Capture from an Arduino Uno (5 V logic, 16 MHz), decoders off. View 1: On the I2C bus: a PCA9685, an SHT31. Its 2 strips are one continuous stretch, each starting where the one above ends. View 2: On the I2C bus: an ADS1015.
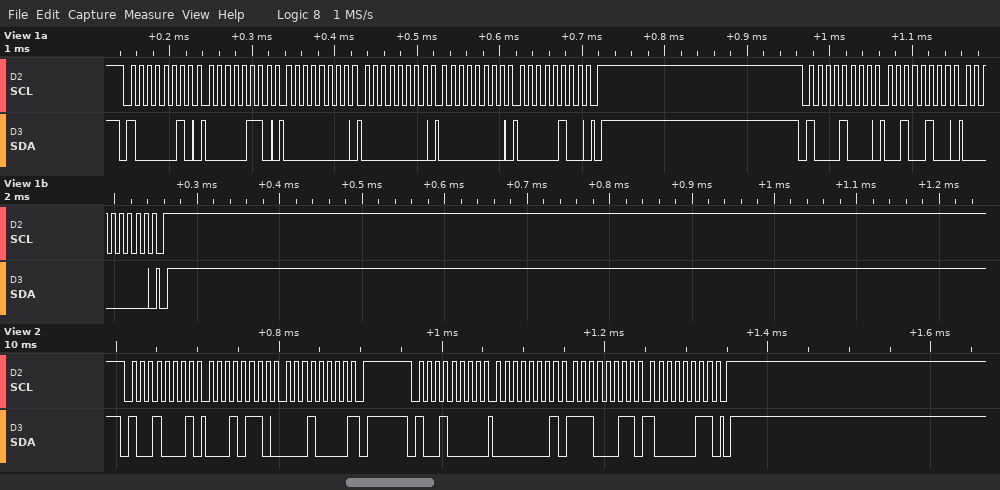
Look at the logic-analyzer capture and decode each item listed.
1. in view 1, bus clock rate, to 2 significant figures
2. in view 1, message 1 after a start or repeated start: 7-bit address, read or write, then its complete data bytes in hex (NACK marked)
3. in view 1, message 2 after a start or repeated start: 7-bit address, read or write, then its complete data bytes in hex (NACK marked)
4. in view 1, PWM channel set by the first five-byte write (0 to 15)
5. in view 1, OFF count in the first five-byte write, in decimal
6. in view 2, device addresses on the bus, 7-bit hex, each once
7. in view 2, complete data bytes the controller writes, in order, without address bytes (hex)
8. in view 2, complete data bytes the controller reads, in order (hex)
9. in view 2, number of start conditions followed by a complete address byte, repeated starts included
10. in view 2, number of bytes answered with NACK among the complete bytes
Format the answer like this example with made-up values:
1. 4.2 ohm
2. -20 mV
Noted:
1. 100 kHz
2. 0x41 write: 06 00 00 00 04
3. 0x44 write: 24 00
4. 0
5. 1024
6. 0x48
7. 01 E3 83
8. 16 10
9. 2
10. 1
